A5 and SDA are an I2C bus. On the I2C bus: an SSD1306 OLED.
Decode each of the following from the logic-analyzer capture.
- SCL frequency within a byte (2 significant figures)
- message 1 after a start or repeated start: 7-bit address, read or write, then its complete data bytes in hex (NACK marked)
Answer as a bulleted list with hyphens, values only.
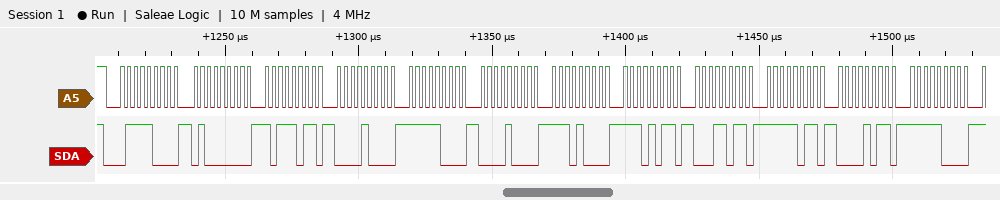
- 400 kHz
- 0x3C write: 40 BB 08 F8 08 E8 EB 1B FB 0B F8
